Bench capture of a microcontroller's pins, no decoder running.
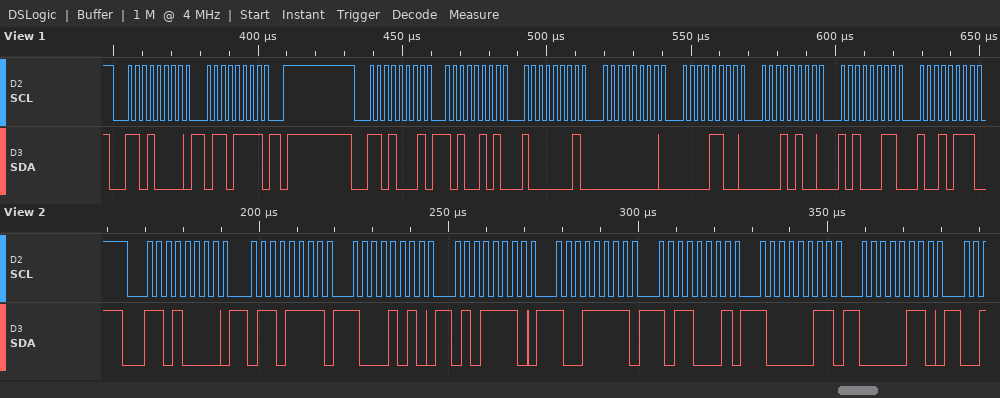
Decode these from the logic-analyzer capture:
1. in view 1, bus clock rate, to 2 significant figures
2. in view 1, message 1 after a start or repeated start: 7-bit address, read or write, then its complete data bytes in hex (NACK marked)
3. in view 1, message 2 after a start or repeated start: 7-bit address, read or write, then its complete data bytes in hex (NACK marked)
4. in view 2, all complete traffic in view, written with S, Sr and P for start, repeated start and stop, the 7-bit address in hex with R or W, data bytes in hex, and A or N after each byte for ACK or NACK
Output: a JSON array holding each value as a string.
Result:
["400 kHz", "0x68 write: 6F", "0x68 read: A5 81 00 0C 14 A3 97", "S 68W A 6F A 8A A 5E A 9F A B1 A 83 A 06 A"]
